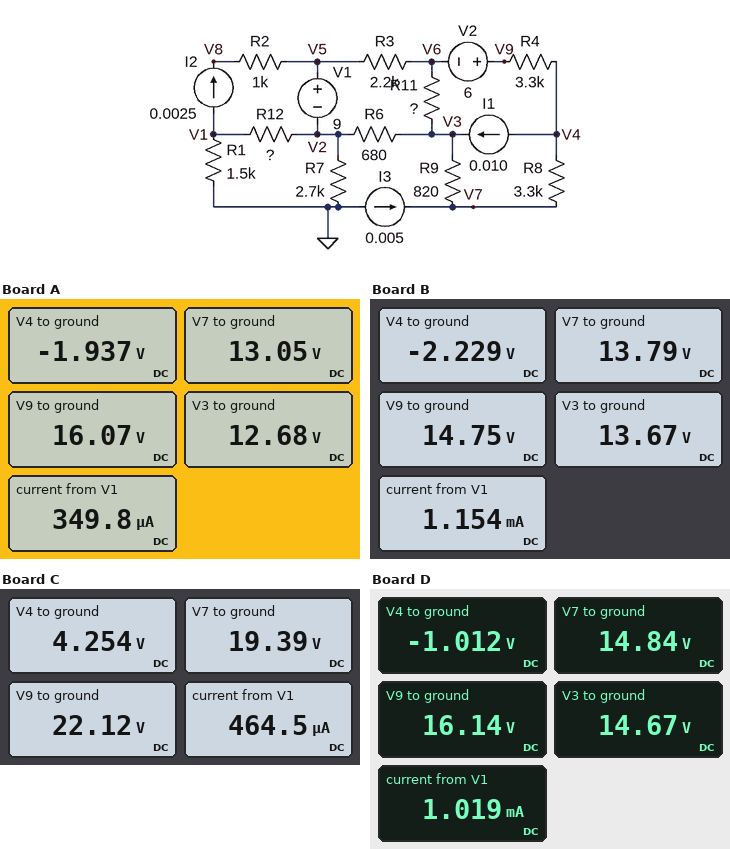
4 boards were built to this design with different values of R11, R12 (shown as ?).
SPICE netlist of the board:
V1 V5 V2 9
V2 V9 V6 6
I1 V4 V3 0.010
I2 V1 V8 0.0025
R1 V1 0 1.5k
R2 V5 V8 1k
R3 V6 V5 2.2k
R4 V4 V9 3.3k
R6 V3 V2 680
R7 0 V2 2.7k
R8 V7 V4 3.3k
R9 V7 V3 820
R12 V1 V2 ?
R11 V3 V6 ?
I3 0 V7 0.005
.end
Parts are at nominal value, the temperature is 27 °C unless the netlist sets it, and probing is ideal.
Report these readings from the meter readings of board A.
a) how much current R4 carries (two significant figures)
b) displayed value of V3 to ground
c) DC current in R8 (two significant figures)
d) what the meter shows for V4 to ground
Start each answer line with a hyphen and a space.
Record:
- 5.5 mA
- 12.68 V
- 4.5 mA
- -1.937 V
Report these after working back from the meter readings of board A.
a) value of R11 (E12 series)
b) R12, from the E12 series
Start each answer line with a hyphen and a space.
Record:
- 1 kΩ
- 820 Ω
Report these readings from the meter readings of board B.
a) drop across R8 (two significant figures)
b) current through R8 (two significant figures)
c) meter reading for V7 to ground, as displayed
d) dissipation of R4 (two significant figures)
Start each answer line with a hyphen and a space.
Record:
- 16 V
- 4.9 mA
- 13.79 V
- 87 mW
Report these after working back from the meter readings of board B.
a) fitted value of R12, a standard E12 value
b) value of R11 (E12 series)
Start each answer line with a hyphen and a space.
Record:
- 1 kΩ
- 3.3 kΩ
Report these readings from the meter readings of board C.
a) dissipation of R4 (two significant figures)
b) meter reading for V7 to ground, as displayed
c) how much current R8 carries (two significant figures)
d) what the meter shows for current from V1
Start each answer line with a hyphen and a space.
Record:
- 97 mW
- 19.39 V
- 4.6 mA
- 464.5 µA
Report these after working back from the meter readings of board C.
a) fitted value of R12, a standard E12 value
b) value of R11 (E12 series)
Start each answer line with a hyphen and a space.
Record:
- 5.6 kΩ
- 1.2 kΩ
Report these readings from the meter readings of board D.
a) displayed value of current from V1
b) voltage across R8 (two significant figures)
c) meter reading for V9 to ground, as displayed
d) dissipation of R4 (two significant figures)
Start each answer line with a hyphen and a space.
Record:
- 1.019 mA
- 16 V
- 16.14 V
- 89 mW
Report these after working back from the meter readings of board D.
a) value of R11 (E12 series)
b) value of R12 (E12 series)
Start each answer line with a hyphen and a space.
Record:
- 2.7 kΩ
- 1.5 kΩ
